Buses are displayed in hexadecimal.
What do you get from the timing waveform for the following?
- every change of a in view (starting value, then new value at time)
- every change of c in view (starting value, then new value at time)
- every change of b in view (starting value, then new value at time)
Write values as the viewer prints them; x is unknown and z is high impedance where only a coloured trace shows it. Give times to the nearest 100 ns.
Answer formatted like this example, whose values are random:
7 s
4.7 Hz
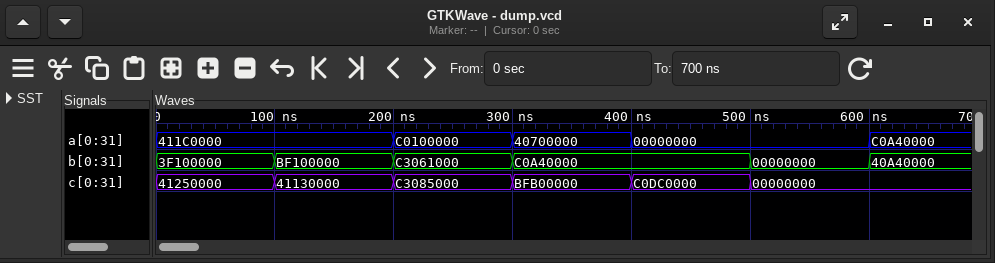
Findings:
411C0000, C0100000 at 200 ns, 40700000 at 300 ns, 00000000 at 400 ns, C0A40000 at 600 ns
41250000, 41130000 at 100 ns, C3085000 at 200 ns, BFB00000 at 300 ns, C0DC0000 at 400 ns, 00000000 at 500 ns
3F100000, BF100000 at 100 ns, C3061000 at 200 ns, C0A40000 at 300 ns, 00000000 at 500 ns, 40A40000 at 600 ns
